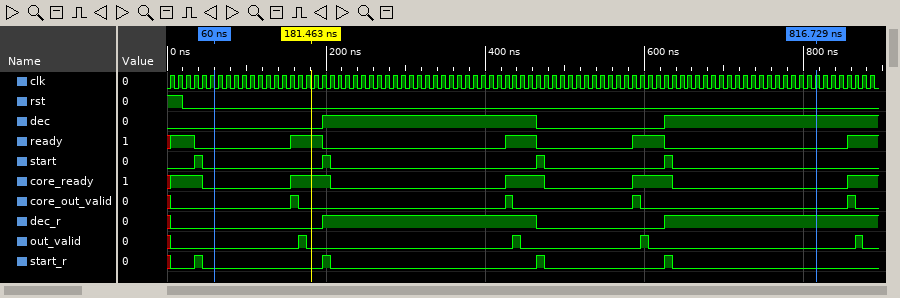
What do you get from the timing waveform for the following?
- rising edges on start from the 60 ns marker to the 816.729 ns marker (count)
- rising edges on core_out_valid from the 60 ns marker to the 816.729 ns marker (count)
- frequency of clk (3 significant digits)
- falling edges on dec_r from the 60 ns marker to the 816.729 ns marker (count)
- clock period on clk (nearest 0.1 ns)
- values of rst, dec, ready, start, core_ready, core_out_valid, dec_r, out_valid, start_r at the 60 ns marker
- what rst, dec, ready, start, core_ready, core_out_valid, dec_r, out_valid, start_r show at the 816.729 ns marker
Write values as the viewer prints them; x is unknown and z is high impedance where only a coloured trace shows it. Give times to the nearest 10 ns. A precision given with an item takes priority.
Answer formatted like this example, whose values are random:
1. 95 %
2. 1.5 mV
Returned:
1. 3
2. 3
3. 100 MHz
4. 1
5. 10 ns
6. rst=0, dec=0, ready=0, start=0, core_ready=0, core_out_valid=0, dec_r=0, out_valid=0, start_r=0
7. rst=0, dec=1, ready=0, start=0, core_ready=0, core_out_valid=0, dec_r=1, out_valid=0, start_r=0
